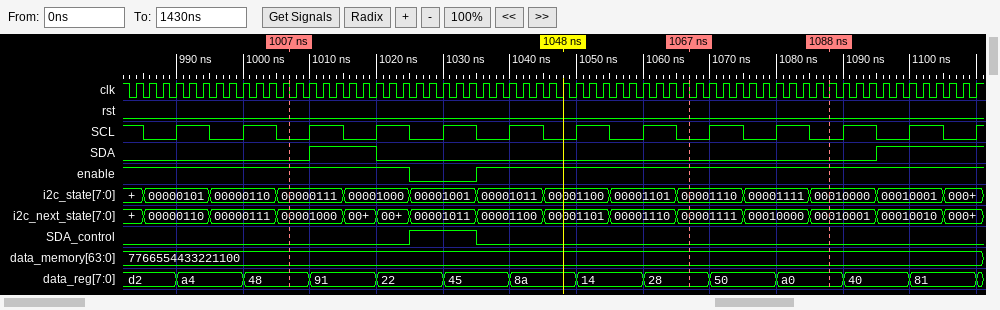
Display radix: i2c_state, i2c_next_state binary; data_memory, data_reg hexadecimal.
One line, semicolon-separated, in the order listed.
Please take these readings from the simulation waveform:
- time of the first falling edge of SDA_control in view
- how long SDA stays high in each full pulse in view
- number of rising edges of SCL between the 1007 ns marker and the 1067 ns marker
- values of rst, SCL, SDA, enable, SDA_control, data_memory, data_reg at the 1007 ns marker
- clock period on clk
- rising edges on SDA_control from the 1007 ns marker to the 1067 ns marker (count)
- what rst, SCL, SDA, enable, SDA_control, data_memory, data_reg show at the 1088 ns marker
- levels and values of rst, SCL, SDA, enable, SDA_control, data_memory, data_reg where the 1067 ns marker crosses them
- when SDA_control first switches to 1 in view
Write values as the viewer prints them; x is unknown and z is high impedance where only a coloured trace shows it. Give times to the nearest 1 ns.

1035 ns; 10 ns; 6; rst=0, SCL=0, SDA=0, enable=1, SDA_control=0, data_memory=7766554433221100, data_reg=48; 2 ns; 1; rst=0, SCL=0, SDA=0, enable=1, SDA_control=0, data_memory=7766554433221100, data_reg=a0; rst=0, SCL=0, SDA=0, enable=1, SDA_control=0, data_memory=7766554433221100, data_reg=28; 1025 ns
